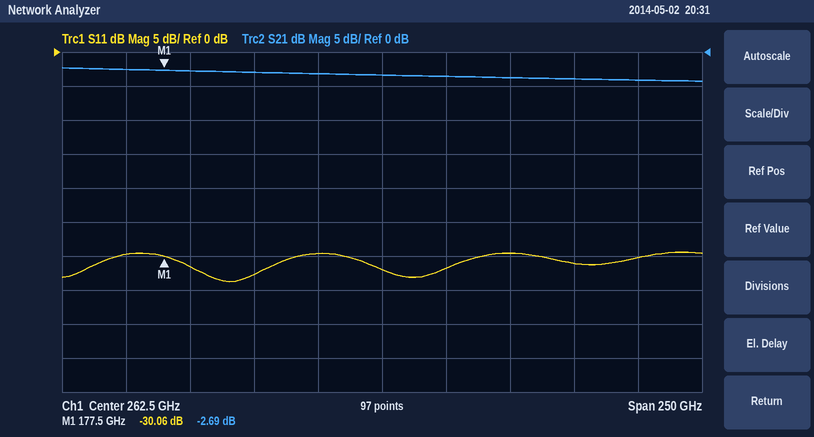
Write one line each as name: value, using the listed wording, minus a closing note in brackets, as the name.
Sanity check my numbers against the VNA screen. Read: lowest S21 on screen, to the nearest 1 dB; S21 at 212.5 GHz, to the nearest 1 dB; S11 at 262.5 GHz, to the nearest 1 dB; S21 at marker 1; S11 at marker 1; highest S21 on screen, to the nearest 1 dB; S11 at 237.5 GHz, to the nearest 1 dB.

lowest S21 on screen, to the nearest 1 dB: -4 dB
S21 at 212.5 GHz, to the nearest 1 dB: -3 dB
S11 at 262.5 GHz, to the nearest 1 dB: -32 dB
S21 at marker 1: -2.69 dB
S11 at marker 1: -30.06 dB
highest S21 on screen, to the nearest 1 dB: -2 dB
S11 at 237.5 GHz, to the nearest 1 dB: -30 dB
